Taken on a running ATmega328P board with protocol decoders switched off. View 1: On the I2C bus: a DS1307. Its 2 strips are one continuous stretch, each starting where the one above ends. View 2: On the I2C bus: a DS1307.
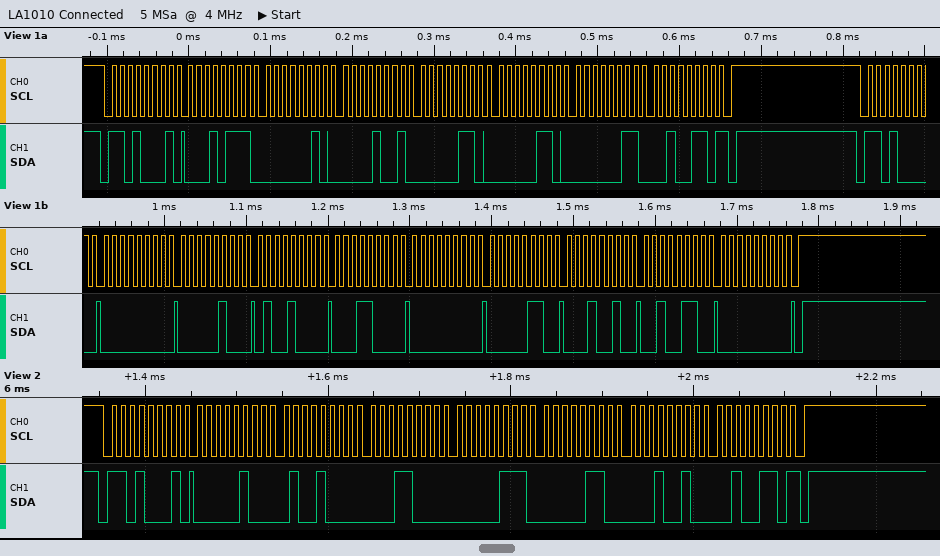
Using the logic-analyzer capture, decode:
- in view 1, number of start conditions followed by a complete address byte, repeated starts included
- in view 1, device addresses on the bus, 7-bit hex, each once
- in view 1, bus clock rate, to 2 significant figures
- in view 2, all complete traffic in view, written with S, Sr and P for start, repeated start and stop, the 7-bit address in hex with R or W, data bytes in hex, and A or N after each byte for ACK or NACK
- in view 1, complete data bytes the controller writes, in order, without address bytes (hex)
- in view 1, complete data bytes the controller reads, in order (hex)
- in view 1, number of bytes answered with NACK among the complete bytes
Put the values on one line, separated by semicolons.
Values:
2; 0x68; 100 kHz; S 68R A 04 A 48 A 18 A 07 A 06 A 12 A 26 N P; 00 04 48 18 00 06 12 26 00; 17 02 09 06 06 03 26; 1
